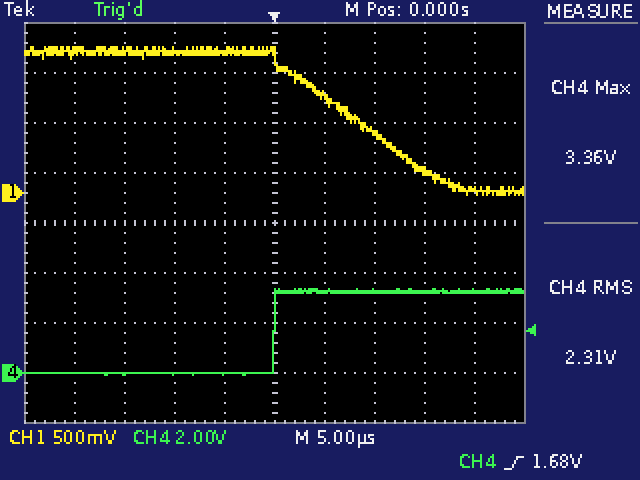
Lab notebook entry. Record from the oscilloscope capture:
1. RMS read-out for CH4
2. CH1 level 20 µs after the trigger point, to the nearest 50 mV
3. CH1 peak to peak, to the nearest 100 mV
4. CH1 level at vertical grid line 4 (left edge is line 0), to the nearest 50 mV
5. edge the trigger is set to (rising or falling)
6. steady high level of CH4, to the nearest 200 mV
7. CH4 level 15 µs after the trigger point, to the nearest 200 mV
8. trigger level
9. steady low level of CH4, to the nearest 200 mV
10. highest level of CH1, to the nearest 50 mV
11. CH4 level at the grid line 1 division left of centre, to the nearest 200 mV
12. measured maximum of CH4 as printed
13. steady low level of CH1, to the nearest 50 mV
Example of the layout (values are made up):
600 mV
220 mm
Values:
2.31 V
0 mV
1.50 V
1.40 V
rising
3.2 V
3.2 V
1.68 V
0.0 V
1.45 V
0.0 V
3.36 V
0 mV
